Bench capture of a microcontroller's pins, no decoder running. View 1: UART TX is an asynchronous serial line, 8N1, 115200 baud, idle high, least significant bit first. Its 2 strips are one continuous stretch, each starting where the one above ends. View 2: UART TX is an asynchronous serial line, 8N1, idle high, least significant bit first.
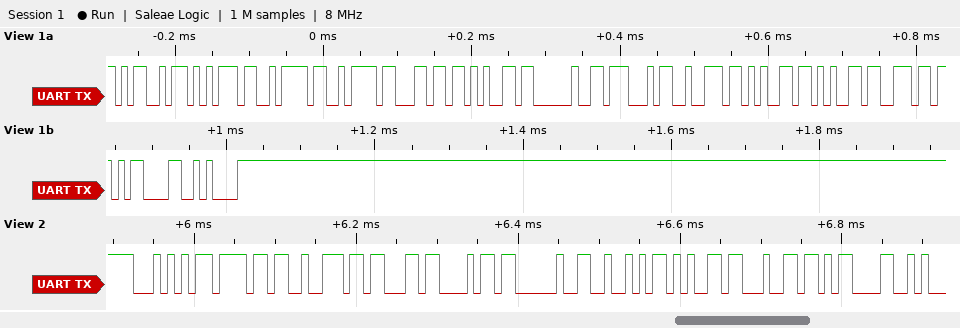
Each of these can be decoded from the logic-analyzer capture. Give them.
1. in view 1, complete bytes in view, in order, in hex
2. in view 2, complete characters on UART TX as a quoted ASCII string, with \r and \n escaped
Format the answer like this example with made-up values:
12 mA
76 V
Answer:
4D 75 7A 7A 6C 65 20 47 72 65 65 6E 0D 0A
"Torch Red\r"
